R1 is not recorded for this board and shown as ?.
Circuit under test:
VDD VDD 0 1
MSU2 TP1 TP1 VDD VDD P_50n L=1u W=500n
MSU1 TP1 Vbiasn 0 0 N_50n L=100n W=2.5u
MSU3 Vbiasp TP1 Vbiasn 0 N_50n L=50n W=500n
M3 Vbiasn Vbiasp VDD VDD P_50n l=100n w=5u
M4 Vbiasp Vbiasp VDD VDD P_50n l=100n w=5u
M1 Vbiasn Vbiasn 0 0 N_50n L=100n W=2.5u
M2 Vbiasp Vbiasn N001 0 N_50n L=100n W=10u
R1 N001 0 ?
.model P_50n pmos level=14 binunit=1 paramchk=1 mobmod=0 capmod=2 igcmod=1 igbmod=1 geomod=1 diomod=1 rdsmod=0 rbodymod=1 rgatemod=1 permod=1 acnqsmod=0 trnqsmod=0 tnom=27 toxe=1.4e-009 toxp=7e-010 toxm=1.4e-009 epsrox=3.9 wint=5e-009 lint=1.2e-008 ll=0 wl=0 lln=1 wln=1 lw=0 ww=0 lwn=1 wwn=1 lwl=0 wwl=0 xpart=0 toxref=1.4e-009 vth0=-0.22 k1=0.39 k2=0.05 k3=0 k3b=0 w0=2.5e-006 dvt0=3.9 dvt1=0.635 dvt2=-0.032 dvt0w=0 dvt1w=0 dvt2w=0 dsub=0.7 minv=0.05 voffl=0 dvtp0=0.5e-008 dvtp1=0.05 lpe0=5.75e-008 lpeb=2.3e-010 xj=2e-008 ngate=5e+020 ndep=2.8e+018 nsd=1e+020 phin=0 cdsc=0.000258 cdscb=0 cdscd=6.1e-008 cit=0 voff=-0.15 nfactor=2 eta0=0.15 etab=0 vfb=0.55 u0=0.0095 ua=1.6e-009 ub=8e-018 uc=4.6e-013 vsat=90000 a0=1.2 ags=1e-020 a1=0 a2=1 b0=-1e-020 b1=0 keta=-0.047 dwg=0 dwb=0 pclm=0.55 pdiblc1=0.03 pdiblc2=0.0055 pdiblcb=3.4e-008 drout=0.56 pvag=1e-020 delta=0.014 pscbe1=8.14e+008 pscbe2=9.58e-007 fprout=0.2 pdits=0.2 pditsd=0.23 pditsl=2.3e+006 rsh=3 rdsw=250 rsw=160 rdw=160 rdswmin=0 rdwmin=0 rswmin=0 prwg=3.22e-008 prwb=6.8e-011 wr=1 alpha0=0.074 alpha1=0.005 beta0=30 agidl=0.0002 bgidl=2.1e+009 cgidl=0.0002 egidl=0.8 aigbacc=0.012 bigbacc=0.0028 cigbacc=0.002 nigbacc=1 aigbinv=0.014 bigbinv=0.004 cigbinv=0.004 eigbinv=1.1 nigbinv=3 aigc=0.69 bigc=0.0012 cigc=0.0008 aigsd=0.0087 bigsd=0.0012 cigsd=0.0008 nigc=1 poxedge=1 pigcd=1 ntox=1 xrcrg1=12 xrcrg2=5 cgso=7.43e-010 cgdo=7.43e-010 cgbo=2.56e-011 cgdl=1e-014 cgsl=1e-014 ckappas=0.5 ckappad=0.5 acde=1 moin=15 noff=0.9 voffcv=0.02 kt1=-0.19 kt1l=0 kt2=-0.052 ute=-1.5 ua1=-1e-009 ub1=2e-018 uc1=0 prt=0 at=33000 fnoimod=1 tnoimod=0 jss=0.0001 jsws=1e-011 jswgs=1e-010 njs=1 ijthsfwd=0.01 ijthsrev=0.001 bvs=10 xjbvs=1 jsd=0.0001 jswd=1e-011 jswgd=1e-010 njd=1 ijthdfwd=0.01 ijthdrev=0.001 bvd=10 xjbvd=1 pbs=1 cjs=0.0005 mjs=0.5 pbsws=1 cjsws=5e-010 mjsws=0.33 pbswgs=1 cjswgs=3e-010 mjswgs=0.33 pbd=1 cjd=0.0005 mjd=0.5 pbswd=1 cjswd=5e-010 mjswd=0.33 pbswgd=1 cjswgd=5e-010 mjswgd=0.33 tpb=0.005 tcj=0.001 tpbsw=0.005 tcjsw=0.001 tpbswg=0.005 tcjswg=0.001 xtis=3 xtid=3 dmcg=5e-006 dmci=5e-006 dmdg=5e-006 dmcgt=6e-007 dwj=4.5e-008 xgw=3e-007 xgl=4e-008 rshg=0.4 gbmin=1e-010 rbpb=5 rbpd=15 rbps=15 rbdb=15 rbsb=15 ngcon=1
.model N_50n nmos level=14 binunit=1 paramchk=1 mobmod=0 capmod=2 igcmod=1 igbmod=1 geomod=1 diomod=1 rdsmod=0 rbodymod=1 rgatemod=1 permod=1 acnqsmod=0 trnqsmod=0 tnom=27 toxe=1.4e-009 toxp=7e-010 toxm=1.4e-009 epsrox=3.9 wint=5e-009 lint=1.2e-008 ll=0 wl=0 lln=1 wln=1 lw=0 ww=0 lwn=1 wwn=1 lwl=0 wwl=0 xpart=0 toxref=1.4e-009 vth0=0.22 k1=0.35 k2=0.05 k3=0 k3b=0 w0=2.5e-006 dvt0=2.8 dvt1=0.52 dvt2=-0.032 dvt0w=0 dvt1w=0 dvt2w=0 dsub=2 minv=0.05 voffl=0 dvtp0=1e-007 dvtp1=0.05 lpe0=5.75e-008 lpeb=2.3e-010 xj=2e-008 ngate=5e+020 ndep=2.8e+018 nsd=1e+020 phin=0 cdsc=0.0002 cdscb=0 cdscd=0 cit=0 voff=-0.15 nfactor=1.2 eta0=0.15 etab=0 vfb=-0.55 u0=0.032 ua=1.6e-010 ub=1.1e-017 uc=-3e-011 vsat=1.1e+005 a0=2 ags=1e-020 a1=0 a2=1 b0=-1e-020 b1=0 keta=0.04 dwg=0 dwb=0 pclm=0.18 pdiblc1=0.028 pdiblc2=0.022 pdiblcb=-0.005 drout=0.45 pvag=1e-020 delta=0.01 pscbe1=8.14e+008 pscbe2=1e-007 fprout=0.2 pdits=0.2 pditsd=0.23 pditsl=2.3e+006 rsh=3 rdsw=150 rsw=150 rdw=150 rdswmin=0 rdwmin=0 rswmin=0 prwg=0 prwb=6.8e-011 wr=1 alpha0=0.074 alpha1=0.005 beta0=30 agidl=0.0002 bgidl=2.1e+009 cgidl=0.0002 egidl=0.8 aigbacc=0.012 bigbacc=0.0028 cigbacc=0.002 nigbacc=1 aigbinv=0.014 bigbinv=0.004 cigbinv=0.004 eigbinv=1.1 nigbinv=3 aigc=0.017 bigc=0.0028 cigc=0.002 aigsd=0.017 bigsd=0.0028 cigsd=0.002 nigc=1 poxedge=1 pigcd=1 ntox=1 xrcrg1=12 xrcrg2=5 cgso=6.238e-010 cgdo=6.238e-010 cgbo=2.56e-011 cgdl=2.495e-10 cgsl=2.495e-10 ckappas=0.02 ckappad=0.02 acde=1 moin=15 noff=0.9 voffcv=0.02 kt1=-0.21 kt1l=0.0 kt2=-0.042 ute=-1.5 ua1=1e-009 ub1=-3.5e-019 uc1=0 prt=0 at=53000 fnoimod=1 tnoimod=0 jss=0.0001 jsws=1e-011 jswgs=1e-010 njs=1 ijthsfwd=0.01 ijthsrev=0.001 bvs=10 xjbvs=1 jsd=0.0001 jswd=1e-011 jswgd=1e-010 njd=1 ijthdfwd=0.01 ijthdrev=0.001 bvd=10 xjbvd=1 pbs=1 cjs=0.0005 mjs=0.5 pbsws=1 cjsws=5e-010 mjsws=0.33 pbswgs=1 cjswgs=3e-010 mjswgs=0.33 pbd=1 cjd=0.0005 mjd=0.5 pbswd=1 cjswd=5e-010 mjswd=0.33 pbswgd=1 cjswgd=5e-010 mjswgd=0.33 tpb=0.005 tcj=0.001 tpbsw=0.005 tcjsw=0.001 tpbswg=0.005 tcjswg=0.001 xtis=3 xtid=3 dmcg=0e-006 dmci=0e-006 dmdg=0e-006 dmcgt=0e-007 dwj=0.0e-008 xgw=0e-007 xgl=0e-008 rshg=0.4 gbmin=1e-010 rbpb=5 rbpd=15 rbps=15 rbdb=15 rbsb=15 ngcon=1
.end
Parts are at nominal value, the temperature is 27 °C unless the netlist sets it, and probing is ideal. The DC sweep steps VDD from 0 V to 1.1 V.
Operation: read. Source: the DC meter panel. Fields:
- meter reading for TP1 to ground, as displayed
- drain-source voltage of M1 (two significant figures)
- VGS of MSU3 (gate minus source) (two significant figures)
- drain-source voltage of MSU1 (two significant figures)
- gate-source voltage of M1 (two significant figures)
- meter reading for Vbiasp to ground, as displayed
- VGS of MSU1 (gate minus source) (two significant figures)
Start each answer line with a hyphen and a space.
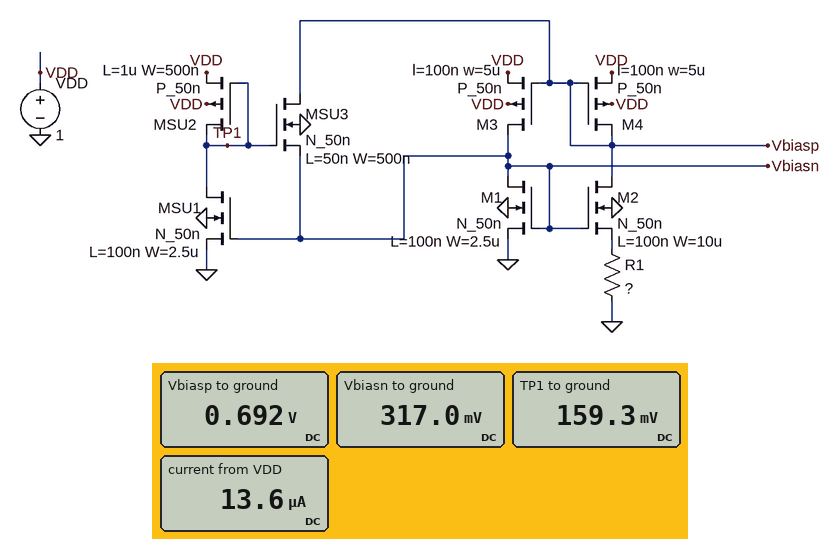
- 159.3 mV
- 320 mV
- -160 mV
- 160 mV
- 320 mV
- 0.692 V
- 320 mV
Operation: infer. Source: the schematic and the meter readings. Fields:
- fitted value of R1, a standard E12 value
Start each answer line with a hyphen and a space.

- 15 kΩ
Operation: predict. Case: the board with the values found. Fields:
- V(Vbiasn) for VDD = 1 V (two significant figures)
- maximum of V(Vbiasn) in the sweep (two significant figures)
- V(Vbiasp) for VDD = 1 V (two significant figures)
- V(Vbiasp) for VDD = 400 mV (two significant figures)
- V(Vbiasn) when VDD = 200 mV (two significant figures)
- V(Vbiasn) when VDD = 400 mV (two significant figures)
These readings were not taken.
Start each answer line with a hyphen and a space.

- 320 mV
- 320 mV
- 690 mV
- 120 mV
- 170 mV
- 280 mV
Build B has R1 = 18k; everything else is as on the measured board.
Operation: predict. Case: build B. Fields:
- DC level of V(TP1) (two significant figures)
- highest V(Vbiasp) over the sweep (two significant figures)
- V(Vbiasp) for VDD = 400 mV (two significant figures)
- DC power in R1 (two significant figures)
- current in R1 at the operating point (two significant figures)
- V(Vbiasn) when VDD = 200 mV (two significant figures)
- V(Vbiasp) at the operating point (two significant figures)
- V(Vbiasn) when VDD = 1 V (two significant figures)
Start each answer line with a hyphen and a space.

- 220 mV
- 800 mV
- 130 mV
- 230 nW
- 3.6 µA
- 170 mV
- 700 mV
- 310 mV
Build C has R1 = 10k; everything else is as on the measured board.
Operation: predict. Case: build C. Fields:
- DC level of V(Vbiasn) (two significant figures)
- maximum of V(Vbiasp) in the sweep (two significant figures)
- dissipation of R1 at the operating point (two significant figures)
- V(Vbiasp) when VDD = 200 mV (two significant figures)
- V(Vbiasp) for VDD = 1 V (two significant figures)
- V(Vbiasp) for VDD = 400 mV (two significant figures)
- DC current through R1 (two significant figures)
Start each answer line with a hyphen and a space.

- 340 mV
- 770 mV
- 430 nW
- 20 mV
- 670 mV
- 100 mV
- 6.5 µA
